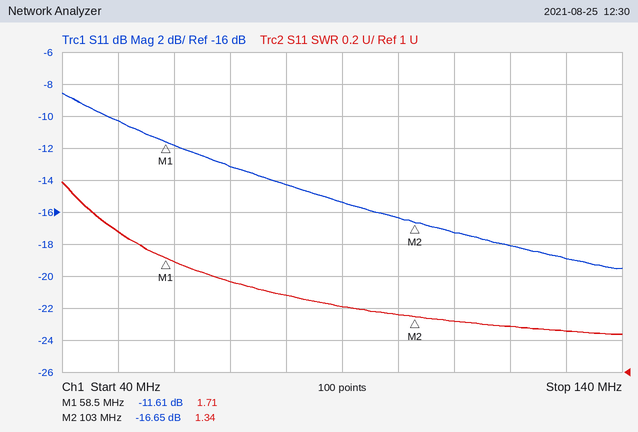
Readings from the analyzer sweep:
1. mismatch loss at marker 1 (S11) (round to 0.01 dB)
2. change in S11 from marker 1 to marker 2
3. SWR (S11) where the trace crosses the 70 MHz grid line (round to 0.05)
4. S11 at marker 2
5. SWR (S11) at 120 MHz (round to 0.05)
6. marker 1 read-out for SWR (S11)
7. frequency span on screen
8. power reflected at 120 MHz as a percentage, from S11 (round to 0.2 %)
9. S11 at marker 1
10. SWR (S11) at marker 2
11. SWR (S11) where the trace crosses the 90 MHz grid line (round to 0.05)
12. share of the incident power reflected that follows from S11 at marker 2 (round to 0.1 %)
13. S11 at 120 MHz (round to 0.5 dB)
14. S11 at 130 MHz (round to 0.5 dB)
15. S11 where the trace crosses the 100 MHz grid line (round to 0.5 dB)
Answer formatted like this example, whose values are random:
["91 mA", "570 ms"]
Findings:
["0.31 dB", "-5.04 dB", "1.55", "-16.65 dB", "1.30", "1.71", "100 MHz", "1.6 %", "-11.61 dB", "1.34", "1.40", "2.2 %", "-18.0 dB", "-19.0 dB", "-16.5 dB"]
